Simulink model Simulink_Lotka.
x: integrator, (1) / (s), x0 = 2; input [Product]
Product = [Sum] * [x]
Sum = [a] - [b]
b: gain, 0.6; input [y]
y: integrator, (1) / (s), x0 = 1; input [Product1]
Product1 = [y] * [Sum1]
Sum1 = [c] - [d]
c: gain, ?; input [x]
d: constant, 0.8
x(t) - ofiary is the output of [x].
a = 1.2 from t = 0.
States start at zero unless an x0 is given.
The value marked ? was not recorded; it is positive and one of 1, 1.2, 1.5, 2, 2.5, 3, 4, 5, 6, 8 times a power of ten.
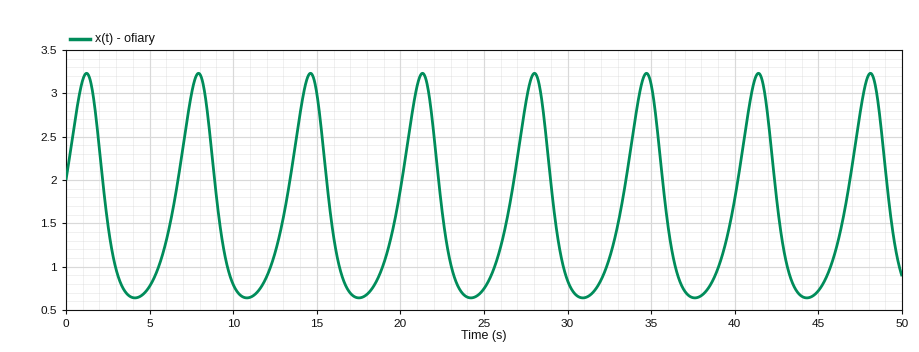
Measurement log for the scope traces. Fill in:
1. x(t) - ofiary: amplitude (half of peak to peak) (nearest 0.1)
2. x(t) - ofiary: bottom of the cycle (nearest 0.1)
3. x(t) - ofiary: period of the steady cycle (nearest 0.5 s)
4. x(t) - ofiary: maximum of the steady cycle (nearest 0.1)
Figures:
1.3
0.6
6.5 s
3.2
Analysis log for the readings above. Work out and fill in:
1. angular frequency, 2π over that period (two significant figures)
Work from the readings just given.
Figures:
0.97 rad/s
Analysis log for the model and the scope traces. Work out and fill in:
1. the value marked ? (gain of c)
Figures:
0.5
